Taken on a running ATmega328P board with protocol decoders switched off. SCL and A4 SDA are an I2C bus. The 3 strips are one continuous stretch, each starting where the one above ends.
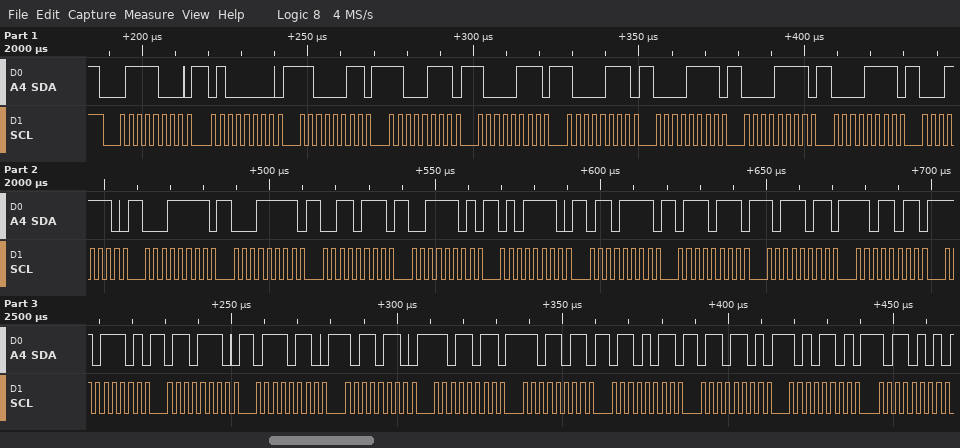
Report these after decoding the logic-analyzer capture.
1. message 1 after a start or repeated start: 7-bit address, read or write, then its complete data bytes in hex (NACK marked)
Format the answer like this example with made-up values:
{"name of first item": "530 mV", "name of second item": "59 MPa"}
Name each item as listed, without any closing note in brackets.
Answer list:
{"message 1 after a start or repeated start: 7-bit address, read or write, then its complete data bytes in hex": "0x3C write: 40 C3 C7 87 87 0F 0F 0F 1E 1F 1F 37 3D 5E 6F 77 BB DB DD 6E 76 B6 DB DB 6B 6D AD B5"}
